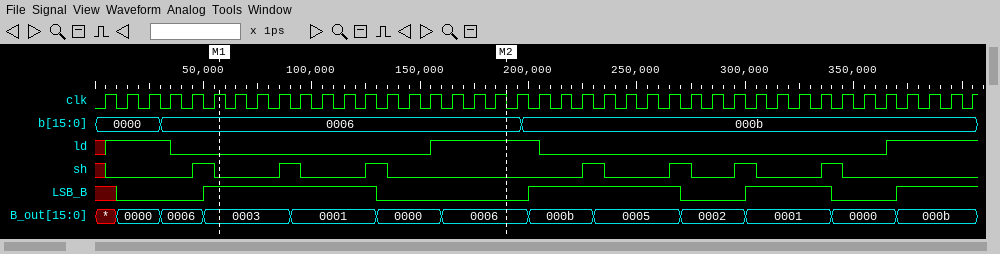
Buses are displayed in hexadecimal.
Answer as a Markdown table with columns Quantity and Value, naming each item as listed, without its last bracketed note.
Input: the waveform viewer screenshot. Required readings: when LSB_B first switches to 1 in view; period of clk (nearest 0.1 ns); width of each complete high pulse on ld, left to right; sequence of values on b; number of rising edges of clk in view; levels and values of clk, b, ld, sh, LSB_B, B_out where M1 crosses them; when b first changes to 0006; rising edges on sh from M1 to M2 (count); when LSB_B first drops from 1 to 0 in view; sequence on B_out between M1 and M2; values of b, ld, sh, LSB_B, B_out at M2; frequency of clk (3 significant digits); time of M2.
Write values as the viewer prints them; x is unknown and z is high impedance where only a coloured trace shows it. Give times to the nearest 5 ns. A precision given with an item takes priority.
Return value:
| Quantity | Value |
|---|---|
| when LSB_B first switches to 1 in view | 50 ns |
| period of clk | 10 ns |
| width of each complete high pulse on ld, left to right | 50 ns |
| sequence of values on b | 0000, 0006, 000b |
| number of rising edges of clk in view | 41 |
| levels and values of clk, b, ld, sh, LSB_B, B_out where M1 crosses them | clk=1, b=0006, ld=0, sh=0, LSB_B=1, B_out=0003 |
| when b first changes to 0006 | 30 ns |
| rising edges on sh from M1 to M2 | 2 |
| when LSB_B first drops from 1 to 0 in view | 130 ns |
| sequence on B_out between M1 and M2 | 0003, 0001, 0000, 0006 |
| values of b, ld, sh, LSB_B, B_out at M2 | b=0006, ld=1, sh=0, LSB_B=0, B_out=0006 |
| frequency of clk | 100 MHz |
| time of M2 | 190 ns |
